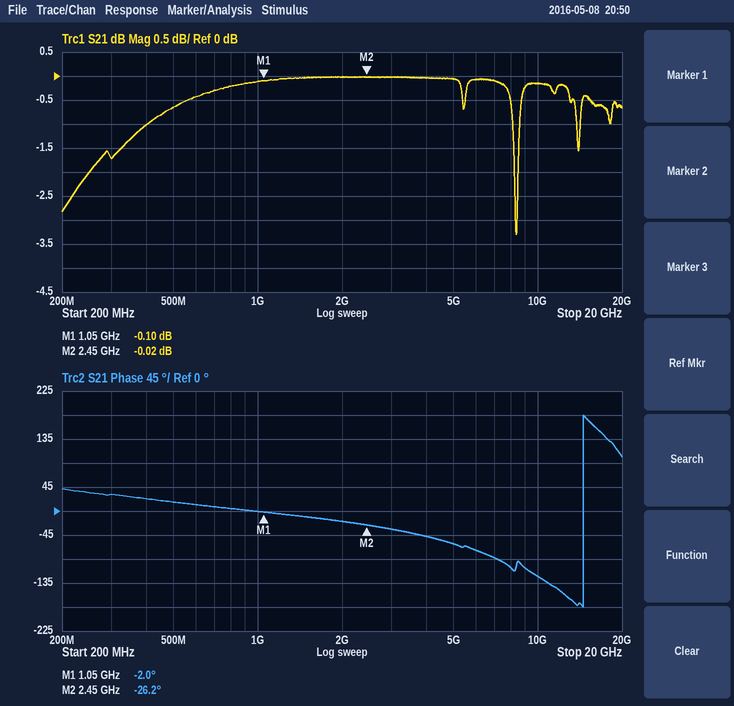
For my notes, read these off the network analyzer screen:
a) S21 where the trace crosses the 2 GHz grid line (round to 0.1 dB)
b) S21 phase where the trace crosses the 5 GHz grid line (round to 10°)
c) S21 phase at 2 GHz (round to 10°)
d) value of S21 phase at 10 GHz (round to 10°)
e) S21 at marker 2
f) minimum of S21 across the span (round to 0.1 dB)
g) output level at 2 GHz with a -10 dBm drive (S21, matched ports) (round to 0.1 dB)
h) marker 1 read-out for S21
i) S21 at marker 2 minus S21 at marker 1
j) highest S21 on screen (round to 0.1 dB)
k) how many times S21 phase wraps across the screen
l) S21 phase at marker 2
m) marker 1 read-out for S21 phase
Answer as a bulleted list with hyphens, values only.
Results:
- 0.0 dB
- -60°
- -20°
- -120°
- -0.02 dB
- -3.3 dB
- -10.0 dBm
- -0.10 dB
- 0.08 dB
- 0.0 dB
- 1
- -26.2°
- -2.0°
